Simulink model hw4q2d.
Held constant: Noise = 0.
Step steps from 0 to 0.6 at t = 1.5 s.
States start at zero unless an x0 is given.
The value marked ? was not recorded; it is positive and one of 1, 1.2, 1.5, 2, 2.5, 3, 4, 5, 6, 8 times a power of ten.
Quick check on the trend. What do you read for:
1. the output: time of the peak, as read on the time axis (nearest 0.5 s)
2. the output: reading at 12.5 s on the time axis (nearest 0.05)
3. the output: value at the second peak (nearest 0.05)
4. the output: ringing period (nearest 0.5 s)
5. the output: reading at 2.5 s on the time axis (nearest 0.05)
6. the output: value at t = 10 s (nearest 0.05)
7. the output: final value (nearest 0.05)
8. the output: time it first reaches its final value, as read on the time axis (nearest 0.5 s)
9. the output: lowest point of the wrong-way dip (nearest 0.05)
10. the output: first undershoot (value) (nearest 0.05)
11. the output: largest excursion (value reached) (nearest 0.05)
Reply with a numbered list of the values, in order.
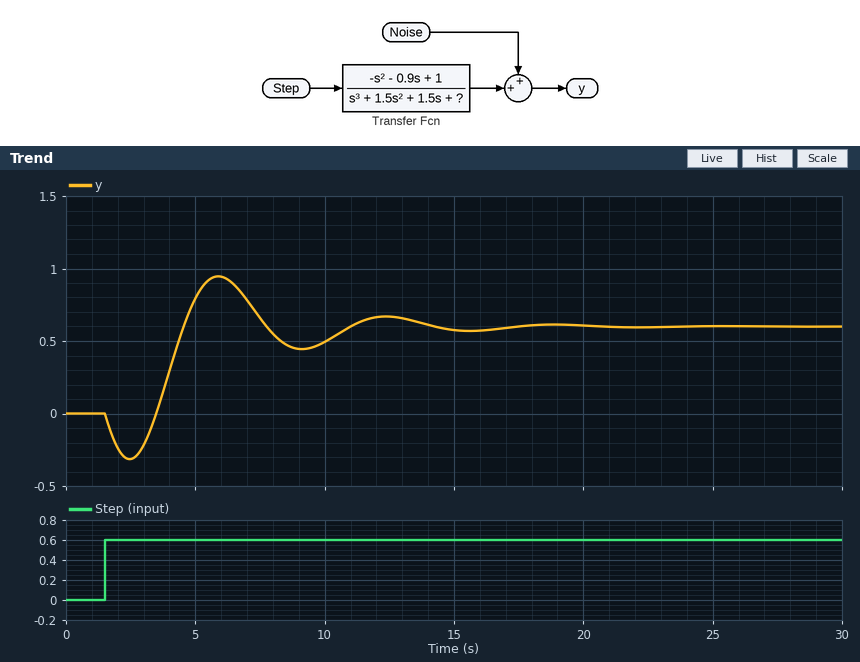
1. 6.0 s
2. 0.65
3. 0.65
4. 6.5 s
5. -0.30
6. 0.50
7. 0.60
8. 4.5 s
9. -0.30
10. 0.45
11. 0.95
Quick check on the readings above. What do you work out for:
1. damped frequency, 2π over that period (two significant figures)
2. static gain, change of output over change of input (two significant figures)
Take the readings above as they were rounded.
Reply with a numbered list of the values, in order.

1. 0.97 rad/s
2. 1.0
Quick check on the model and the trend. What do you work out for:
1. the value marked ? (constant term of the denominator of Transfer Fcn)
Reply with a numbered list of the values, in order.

1. 1
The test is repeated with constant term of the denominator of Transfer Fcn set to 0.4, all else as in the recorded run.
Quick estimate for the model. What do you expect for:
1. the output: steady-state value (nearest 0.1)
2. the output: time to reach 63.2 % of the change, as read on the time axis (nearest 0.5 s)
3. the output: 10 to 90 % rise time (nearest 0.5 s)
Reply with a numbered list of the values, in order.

1. 1.5
2. 5.5 s
3. 5.0 s
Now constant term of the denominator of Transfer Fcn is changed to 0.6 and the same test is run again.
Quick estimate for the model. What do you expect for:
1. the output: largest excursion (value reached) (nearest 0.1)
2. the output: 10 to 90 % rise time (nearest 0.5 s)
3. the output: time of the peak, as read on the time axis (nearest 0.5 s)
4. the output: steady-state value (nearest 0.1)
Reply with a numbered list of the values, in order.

1. 1.1
2. 1.5 s
3. 7.0 s
4. 1.0
